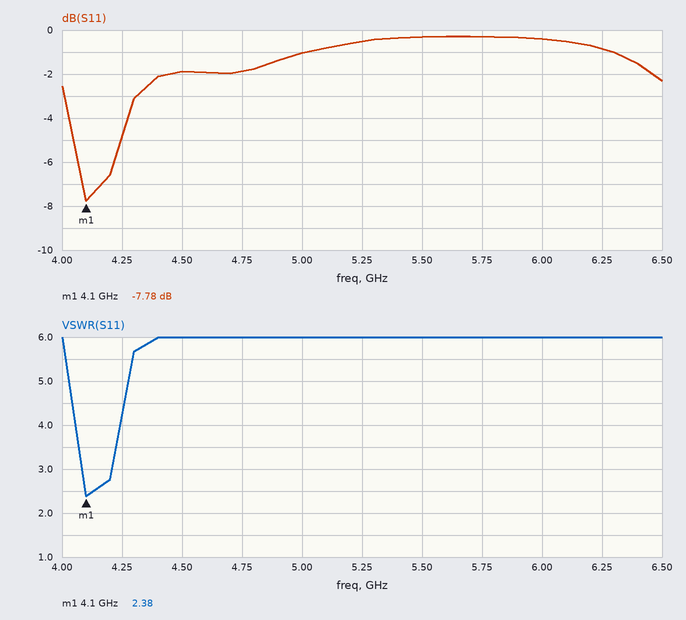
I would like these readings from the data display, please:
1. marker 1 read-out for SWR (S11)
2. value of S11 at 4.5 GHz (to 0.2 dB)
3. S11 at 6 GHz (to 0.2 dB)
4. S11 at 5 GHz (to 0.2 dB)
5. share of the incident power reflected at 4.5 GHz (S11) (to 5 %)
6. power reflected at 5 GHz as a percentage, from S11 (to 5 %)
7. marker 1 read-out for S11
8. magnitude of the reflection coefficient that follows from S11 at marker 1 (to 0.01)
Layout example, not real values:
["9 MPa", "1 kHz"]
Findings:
["2.38", "-1.8 dB", "-0.4 dB", "-1.0 dB", "65 %", "80 %", "-7.78 dB", "0.41"]
